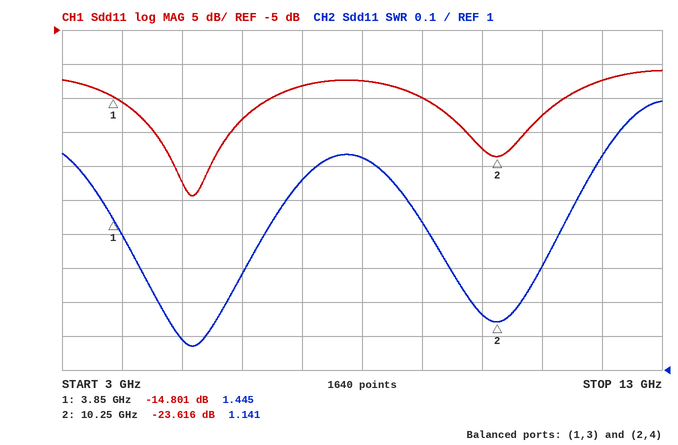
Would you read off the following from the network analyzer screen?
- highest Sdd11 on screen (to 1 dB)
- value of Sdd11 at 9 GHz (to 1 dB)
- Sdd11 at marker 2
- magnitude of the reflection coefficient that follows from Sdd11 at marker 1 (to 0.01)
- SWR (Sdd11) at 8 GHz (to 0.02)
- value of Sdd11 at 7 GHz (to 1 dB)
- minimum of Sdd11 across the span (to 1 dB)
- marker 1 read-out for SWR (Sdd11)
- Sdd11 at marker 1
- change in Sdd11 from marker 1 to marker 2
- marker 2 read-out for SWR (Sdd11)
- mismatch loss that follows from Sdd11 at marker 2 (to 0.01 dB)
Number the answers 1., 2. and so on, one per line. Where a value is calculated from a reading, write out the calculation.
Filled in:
1. -11 dB
2. -15 dB
3. -23.616 dB
4. 10^(-14.801/20) ≈ 0.18
5. 1.62
6. -13 dB
7. -29 dB
8. 1.445
9. -14.801 dB
10. -23.616 − (-14.801) = -8.815 dB
11. 1.141
12. −10 log10(1 − 10^(-23.616/10)) ≈ 0.02 dB
